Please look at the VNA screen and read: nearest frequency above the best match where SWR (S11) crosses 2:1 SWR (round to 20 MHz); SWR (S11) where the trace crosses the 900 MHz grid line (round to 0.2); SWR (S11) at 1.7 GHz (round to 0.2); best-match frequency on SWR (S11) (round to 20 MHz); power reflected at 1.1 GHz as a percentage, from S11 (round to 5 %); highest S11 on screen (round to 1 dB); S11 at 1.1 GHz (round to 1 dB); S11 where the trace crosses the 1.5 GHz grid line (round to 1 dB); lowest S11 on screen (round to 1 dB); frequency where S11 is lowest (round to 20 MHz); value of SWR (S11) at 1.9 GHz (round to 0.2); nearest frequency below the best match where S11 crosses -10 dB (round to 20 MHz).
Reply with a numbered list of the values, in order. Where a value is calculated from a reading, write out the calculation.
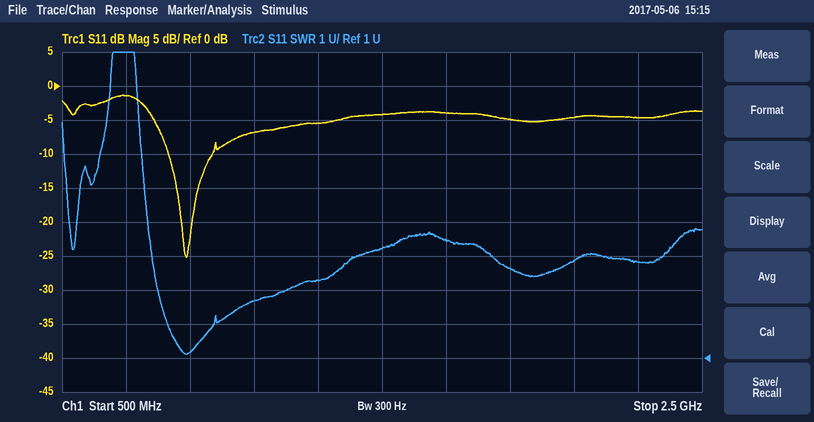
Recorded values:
1. 980 MHz
2. 1.2
3. 4.4
4. 880 MHz
5. 10^(-7/10) ≈ 20 %
6. -1 dB
7. -7 dB
8. -4 dB
9. -25 dB
10. 880 MHz
11. 3.6
12. 840 MHz
